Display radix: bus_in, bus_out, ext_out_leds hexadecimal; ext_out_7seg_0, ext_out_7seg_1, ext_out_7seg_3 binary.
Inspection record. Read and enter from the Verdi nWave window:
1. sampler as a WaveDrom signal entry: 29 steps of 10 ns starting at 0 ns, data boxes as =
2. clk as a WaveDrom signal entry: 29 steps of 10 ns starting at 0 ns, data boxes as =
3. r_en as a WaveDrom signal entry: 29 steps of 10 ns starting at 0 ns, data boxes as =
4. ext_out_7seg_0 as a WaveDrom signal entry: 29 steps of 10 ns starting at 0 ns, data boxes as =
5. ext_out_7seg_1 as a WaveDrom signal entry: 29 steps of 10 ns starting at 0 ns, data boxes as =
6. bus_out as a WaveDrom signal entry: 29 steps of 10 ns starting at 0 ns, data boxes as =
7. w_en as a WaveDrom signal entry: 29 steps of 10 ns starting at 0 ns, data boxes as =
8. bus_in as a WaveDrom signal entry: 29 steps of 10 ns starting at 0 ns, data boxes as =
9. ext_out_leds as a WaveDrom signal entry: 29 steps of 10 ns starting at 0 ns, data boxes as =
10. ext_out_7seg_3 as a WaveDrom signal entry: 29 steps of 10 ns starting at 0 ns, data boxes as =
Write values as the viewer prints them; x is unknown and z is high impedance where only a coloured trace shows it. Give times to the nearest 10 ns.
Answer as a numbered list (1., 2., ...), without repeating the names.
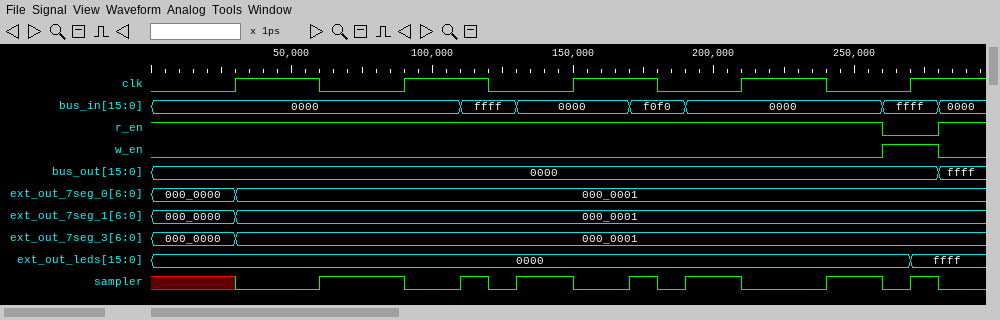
1. {name: 'sampler', wave: 'x..0..1..0.101.0.101.0..1.010'}
2. {name: 'clk', wave: '0..1..0..1..0..1..0..1..0..1.'}
3. {name: 'r_en', wave: '1.........................0.1'}
4. {name: 'ext_out_7seg_0', wave: '=..=.........................', data: '000_0000 000_0001'}
5. {name: 'ext_out_7seg_1', wave: '=..=.........................', data: '000_0000 000_0001'}
6. {name: 'bus_out', wave: '=...........................=', data: '0000 ffff'}
7. {name: 'w_en', wave: '0.........................1.0'}
8. {name: 'bus_in', wave: '=..........=.=...=.=......=.=', data: '0000 ffff 0000 f0f0 0000 ffff 0000'}
9. {name: 'ext_out_leds', wave: '=..........................=.', data: '0000 ffff'}
10. {name: 'ext_out_7seg_3', wave: '=..=.........................', data: '000_0000 000_0001'}
